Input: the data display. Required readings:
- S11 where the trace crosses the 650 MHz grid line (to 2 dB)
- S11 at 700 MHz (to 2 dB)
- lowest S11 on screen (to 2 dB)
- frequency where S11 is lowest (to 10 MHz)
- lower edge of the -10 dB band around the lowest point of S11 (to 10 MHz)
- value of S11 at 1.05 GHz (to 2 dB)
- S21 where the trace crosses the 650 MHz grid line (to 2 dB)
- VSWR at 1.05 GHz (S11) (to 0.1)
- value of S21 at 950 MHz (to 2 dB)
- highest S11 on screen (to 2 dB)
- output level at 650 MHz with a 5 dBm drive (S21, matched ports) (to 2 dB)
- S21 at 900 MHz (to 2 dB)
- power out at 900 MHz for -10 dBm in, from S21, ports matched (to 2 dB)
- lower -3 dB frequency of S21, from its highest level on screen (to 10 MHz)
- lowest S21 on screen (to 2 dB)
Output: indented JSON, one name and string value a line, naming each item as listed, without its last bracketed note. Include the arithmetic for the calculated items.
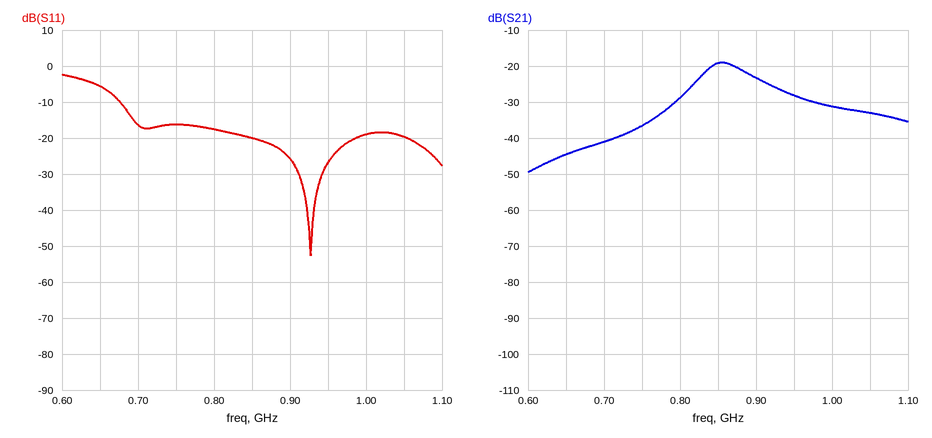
{
  "S11 where the trace crosses the 650 MHz grid line": "-6 dB",
  "S11 at 700 MHz": "-16 dB",
  "lowest S11 on screen": "-52 dB",
  "frequency where S11 is lowest": "930 MHz",
  "lower edge of the -10 dB band around the lowest point of S11": "680 MHz",
  "value of S11 at 1.05 GHz": "-20 dB",
  "S21 where the trace crosses the 650 MHz grid line": "-44 dB",
  "VSWR at 1.05 GHz (S11)": "|Γ| = 10^(-20/20) = 0.1000; VSWR = (1 + 0.1000)/(1 − 0.1000) ≈ 1.2",
  "value of S21 at 950 MHz": "-28 dB",
  "highest S11 on screen": "-2 dB",
  "output level at 650 MHz with a 5 dBm drive (S21, matched ports)": "5 dBm + (-44 dB) = -40 dBm",
  "S21 at 900 MHz": "-24 dB",
  "power out at 900 MHz for -10 dBm in, from S21, ports matched": "-10 dBm + (-24 dB) = -34 dBm",
  "lower -3 dB frequency of S21, from its highest level on screen": "830 MHz",
  "lowest S21 on screen": "-50 dB"
}
